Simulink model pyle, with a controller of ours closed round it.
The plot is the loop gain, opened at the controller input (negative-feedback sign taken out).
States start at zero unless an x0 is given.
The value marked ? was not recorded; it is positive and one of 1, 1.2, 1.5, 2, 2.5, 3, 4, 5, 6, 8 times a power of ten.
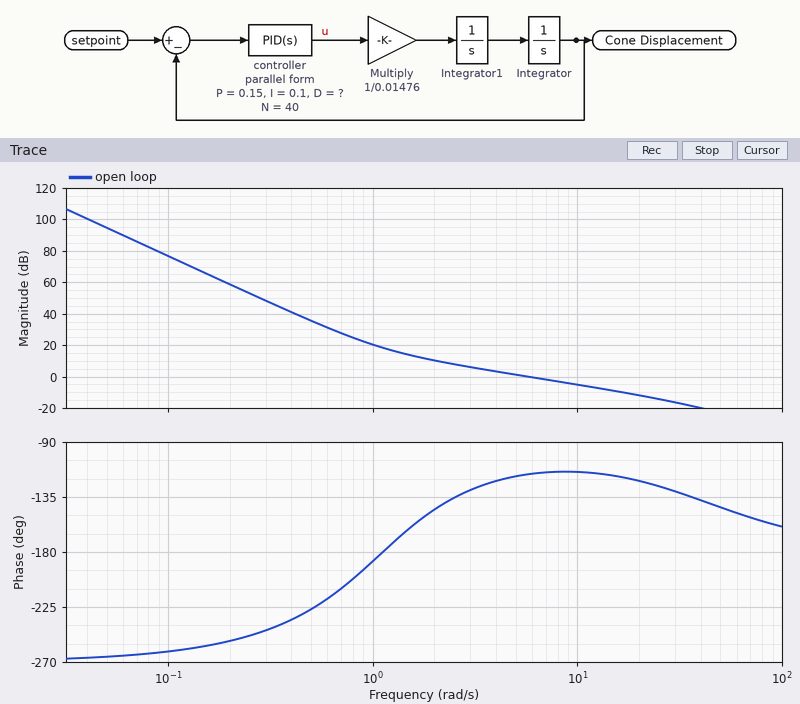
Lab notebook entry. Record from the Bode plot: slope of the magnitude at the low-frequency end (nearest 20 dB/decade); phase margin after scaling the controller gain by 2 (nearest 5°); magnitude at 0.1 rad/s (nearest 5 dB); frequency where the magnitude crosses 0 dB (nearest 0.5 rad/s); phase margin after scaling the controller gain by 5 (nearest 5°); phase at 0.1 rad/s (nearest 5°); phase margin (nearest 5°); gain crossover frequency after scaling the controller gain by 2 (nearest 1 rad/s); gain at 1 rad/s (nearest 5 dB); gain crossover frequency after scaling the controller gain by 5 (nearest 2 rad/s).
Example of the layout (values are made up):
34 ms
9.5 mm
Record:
-60 dB/decade
65°
75 dB
5.5 rad/s
55°
-260°
65°
11 rad/s
20 dB
24 rad/s
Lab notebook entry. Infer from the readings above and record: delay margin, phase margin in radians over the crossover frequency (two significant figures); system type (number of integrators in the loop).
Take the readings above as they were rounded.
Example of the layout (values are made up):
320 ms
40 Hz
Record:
0.21 s
3
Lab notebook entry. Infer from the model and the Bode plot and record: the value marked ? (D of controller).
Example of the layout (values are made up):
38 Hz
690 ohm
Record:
0.08
